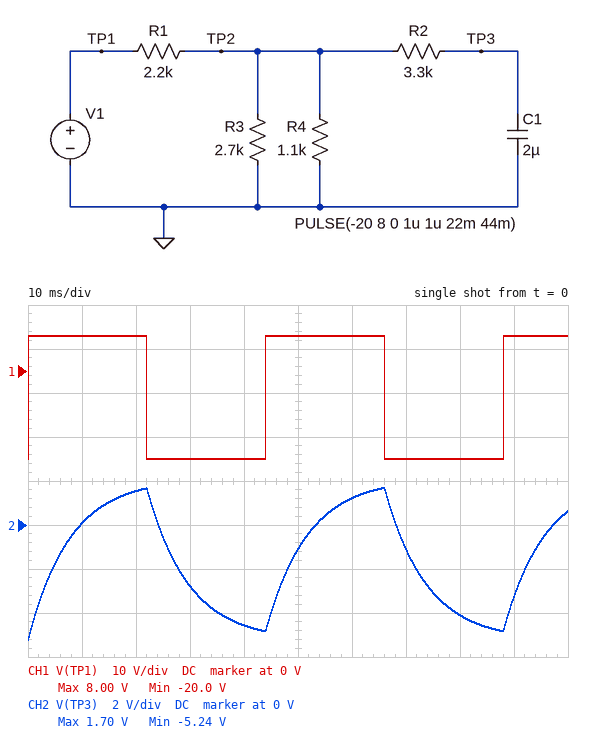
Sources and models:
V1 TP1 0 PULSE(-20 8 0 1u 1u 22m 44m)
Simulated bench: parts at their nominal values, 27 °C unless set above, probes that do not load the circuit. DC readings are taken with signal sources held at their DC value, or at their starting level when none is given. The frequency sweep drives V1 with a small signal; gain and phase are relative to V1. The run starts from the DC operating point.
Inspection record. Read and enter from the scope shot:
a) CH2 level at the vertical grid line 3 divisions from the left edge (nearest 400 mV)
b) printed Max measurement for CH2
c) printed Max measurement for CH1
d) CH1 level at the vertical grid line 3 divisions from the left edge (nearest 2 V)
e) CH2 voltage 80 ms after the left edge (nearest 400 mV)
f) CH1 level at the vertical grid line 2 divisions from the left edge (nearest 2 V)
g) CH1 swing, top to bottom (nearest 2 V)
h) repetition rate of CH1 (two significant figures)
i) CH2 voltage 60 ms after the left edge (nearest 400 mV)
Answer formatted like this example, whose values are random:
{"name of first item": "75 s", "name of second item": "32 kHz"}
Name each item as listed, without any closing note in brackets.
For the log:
{"CH2 level at the vertical grid line 3 divisions from the left edge": "-2.8 V", "printed Max measurement for CH2": "1.70 V", "printed Max measurement for CH1": "8.00 V", "CH1 level at the vertical grid line 3 divisions from the left edge": "-20 V", "CH2 voltage 80 ms after the left edge": "-4.0 V", "CH1 level at the vertical grid line 2 divisions from the left edge": "8 V", "CH1 swing, top to bottom": "28 V", "repetition rate of CH1": "23 Hz", "CH2 voltage 60 ms after the left edge": "1.2 V"}
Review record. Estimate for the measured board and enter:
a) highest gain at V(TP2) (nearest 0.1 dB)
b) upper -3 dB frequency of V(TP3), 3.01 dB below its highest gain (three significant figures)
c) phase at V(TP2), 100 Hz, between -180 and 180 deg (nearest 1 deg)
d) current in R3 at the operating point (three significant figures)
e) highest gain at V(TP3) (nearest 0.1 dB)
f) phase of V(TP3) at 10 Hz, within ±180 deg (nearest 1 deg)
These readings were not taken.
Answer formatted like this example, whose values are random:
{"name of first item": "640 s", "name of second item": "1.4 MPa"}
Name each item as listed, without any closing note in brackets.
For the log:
{"highest gain at V(TP2)": "-11.6 dB", "upper -3 dB frequency of V(TP3), 3.01 dB below its highest gain": "20.5 Hz", "phase at V(TP2), 100 Hz, between -180 and 180 deg": "-2 deg", "current in R3 at the operating point": "1.94 mA", "highest gain at V(TP3)": "-11.6 dB", "phase of V(TP3) at 10 Hz, within ±180 deg": "-26 deg"}
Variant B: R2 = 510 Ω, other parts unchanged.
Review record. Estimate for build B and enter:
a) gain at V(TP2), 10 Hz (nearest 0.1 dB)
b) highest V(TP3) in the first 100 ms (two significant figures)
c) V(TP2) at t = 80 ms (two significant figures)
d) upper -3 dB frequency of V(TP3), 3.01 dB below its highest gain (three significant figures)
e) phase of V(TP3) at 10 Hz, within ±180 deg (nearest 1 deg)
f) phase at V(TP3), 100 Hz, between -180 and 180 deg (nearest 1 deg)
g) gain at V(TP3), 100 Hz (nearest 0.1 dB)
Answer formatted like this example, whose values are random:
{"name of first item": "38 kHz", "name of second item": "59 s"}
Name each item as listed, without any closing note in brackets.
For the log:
{"gain at V(TP2), 10 Hz": "-11.7 dB", "highest V(TP3) in the first 100 ms": "2.1 V", "V(TP2) at t = 80 ms": "-5.2 V", "upper -3 dB frequency of V(TP3), 3.01 dB below its highest gain": "73.2 Hz", "phase of V(TP3) at 10 Hz, within ±180 deg": "-8 deg", "phase at V(TP3), 100 Hz, between -180 and 180 deg": "-54 deg", "gain at V(TP3), 100 Hz": "-16.2 dB"}
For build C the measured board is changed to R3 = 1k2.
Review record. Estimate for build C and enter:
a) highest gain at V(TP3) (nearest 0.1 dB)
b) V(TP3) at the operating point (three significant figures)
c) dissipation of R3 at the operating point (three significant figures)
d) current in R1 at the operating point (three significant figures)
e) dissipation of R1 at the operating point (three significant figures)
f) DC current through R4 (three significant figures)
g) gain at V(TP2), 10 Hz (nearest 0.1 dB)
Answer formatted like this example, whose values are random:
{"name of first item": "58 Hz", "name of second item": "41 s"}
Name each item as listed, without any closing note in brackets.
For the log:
{"highest gain at V(TP3)": "-13.7 dB", "V(TP3) at the operating point": "-4.14 V", "dissipation of R3 at the operating point": "14.3 mW", "current in R1 at the operating point": "7.21 mA", "dissipation of R1 at the operating point": "114 mW", "DC current through R4": "3.76 mA", "gain at V(TP2), 10 Hz": "-13.9 dB"}
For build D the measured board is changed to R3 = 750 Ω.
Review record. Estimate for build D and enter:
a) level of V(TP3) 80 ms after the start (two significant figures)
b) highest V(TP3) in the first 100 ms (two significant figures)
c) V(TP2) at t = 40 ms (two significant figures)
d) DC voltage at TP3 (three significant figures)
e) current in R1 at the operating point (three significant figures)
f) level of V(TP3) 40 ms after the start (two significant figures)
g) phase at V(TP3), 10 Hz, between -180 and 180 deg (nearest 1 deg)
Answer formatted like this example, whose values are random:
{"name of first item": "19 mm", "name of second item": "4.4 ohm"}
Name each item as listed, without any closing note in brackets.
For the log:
{"level of V(TP3) 80 ms after the start": "-2.7 V", "highest V(TP3) in the first 100 ms": "1.1 V", "V(TP2) at t = 40 ms": "-3.3 V", "DC voltage at TP3": "-3.37 V", "current in R1 at the operating point": "7.56 mA", "level of V(TP3) 40 ms after the start": "-3.0 V", "phase at V(TP3), 10 Hz, between -180 and 180 deg": "-25 deg"}
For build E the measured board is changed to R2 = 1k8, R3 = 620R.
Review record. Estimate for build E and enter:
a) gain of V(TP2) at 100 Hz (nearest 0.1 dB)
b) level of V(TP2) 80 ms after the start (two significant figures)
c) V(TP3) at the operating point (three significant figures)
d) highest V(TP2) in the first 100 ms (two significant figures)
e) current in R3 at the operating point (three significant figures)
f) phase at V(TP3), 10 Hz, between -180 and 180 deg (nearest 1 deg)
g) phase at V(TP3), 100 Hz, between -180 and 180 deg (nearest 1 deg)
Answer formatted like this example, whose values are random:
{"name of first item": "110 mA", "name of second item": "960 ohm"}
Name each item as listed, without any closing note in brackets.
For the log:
{"gain of V(TP2) at 100 Hz": "-17.6 dB", "level of V(TP2) 80 ms after the start": "-3.0 V", "V(TP3) at the operating point": "-3.05 V", "highest V(TP2) in the first 100 ms": "1.2 V", "current in R3 at the operating point": "4.93 mA", "phase at V(TP3), 10 Hz, between -180 and 180 deg": "-15 deg", "phase at V(TP3), 100 Hz, between -180 and 180 deg": "-70 deg"}
